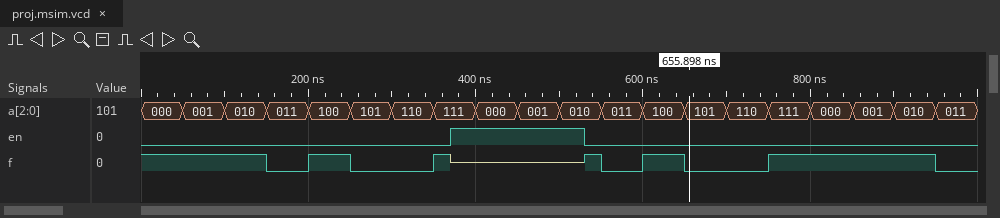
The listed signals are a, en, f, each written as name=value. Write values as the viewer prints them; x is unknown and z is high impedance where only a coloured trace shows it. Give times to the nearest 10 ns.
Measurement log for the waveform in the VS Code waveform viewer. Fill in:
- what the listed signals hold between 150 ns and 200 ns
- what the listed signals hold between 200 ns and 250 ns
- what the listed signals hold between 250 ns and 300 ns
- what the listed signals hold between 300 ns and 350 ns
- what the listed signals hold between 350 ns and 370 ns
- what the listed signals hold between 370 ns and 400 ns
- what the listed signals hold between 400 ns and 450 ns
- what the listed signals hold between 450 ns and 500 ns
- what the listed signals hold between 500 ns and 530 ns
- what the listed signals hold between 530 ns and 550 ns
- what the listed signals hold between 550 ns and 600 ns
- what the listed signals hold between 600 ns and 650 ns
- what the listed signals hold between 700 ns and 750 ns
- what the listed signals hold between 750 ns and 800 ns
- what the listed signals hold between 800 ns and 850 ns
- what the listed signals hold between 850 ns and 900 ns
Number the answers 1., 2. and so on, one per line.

1. a=011, en=0, f=0
2. a=100, en=0, f=1
3. a=101, en=0, f=0
4. a=110, en=0, f=0
5. a=111, en=0, f=1
6. a=111, en=1, f=z
7. a=000, en=1, f=z
8. a=001, en=1, f=z
9. a=010, en=1, f=z
10. a=010, en=0, f=1
11. a=011, en=0, f=0
12. a=100, en=0, f=1
13. a=110, en=0, f=0
14. a=111, en=0, f=1
15. a=000, en=0, f=1
16. a=001, en=0, f=1
